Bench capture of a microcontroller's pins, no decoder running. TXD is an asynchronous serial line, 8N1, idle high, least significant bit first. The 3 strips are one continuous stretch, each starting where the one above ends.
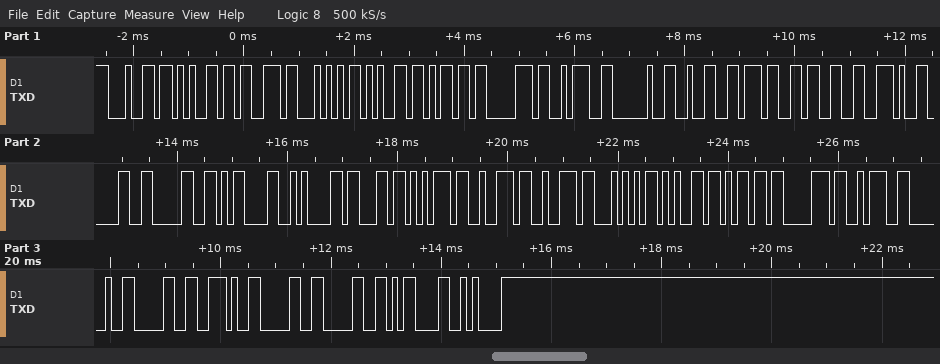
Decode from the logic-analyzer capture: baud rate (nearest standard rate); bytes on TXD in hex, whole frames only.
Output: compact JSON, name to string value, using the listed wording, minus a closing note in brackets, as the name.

{"baud rate": "9600 baud", "bytes on TXD in hex, whole frames only": "0x64 0x65 0x73 0x54 0x65 0x6D 0x70 0x3A 0x20 0x32 0x37 0x33 0x2E 0x30 0x30 0x0D 0x0A 0x63 0x75 0x72 0x72 0x54 0x65 0x6D 0x70 0x3A 0x20 0x30 0x2E 0x30 0x30 0x0D 0x0A"}
